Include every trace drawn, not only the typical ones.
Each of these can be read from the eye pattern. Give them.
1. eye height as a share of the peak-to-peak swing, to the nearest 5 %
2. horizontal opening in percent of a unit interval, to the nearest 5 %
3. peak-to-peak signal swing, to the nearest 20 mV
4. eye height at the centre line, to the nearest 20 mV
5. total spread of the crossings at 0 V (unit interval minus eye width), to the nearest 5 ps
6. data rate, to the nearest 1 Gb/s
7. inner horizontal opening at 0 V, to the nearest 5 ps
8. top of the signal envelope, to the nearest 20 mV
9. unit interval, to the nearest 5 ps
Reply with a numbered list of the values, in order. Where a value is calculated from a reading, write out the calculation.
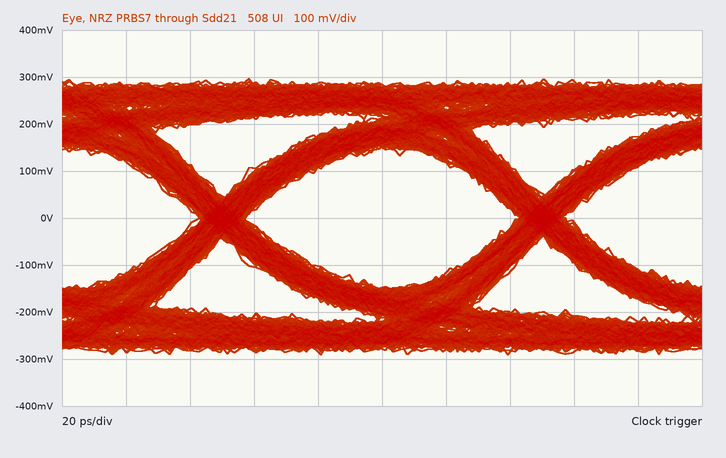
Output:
1. 300 mV / 580 mV ≈ 51.7 %, so 50 % to the nearest 5 %
2. 85 ps / 100 ps ≈ 85 %
3. 580 mV
4. 300 mV
5. 15 ps
6. 10 Gb/s
7. 85 ps
8. 300 mV
9. 100 ps
